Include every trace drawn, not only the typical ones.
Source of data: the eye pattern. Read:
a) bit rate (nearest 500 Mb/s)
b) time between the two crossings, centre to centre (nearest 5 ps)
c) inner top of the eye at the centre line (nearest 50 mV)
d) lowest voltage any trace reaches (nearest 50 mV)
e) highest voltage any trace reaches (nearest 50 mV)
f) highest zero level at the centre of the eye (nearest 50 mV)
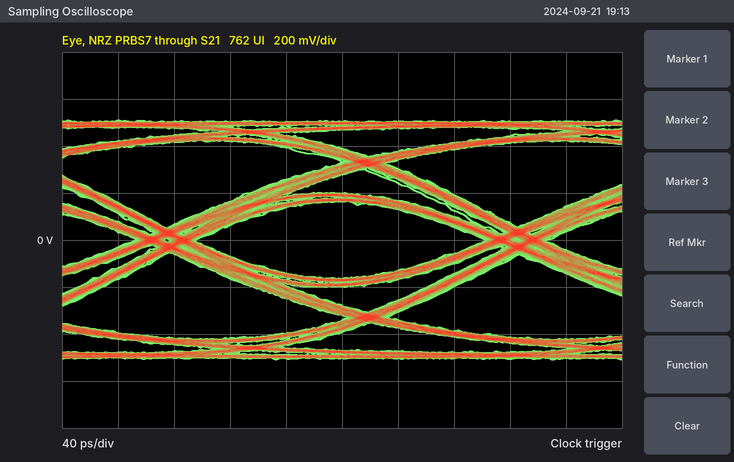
4.0 Gb/s
250 ps
150 mV
-500 mV
500 mV
-150 mV
